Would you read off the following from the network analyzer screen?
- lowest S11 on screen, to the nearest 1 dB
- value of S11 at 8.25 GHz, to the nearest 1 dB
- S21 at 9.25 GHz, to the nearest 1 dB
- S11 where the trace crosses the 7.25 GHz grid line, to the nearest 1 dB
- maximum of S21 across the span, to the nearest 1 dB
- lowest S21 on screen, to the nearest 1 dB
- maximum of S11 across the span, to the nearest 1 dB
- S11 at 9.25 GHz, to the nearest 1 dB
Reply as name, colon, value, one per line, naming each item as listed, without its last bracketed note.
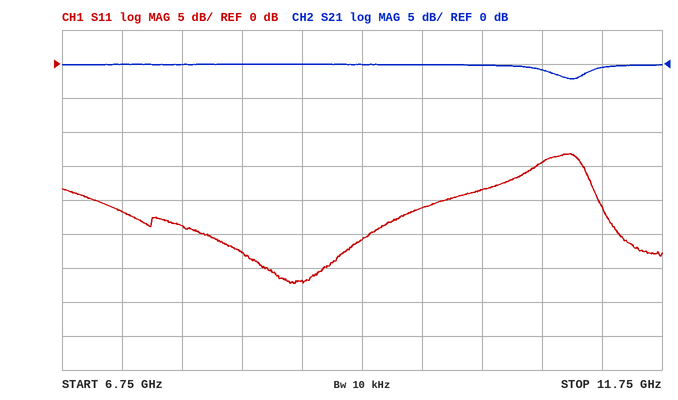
lowest S11 on screen, to the nearest 1 dB: -32 dB
value of S11 at 8.25 GHz, to the nearest 1 dB: -28 dB
S21 at 9.25 GHz, to the nearest 1 dB: 0 dB
S11 where the trace crosses the 7.25 GHz grid line, to the nearest 1 dB: -22 dB
maximum of S21 across the span, to the nearest 1 dB: 0 dB
lowest S21 on screen, to the nearest 1 dB: -2 dB
maximum of S11 across the span, to the nearest 1 dB: -13 dB
S11 at 9.25 GHz, to the nearest 1 dB: -26 dB
